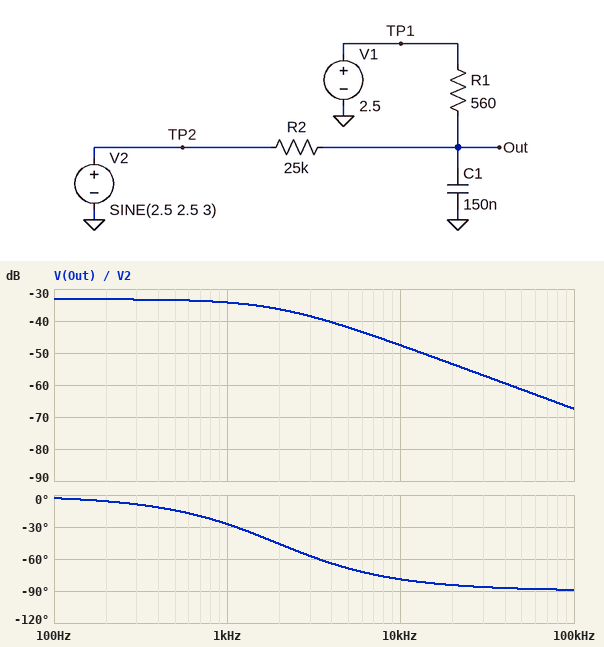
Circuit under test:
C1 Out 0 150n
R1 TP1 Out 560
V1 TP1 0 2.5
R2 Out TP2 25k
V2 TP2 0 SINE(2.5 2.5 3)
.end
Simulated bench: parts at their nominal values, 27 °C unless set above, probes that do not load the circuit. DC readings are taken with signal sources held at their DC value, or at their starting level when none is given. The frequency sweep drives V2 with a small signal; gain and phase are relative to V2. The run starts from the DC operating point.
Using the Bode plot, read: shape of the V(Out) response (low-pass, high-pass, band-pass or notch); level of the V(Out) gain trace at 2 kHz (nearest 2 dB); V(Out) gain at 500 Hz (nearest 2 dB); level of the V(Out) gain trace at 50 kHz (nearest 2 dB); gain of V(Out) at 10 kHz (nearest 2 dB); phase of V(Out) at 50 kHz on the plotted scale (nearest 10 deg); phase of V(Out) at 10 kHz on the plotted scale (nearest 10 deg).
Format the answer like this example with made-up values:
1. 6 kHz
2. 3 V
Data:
1. low-pass
2. -36 dB
3. -34 dB
4. -62 dB
5. -48 dB
6. -90 deg
7. -80 deg
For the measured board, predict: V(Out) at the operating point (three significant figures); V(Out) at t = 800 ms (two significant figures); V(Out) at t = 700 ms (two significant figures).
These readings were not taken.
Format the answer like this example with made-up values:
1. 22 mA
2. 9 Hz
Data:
1. 2.50 V
2. 2.5 V
3. 2.5 V
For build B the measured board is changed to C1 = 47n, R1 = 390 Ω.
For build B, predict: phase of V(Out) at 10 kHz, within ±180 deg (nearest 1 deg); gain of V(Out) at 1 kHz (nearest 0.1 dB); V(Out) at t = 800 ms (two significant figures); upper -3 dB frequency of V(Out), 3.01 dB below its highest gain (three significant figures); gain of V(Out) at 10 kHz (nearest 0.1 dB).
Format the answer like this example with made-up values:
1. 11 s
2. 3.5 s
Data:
1. -49 deg
2. -36.3 dB
3. 2.5 V
4. 8.82 kHz
5. -39.9 dB
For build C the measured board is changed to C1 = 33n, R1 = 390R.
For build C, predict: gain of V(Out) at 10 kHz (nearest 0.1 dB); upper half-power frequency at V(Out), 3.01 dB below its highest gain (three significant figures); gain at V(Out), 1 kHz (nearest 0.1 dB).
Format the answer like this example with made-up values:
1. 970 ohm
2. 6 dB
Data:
1. -38.4 dB
2. 12.6 kHz
3. -36.3 dB
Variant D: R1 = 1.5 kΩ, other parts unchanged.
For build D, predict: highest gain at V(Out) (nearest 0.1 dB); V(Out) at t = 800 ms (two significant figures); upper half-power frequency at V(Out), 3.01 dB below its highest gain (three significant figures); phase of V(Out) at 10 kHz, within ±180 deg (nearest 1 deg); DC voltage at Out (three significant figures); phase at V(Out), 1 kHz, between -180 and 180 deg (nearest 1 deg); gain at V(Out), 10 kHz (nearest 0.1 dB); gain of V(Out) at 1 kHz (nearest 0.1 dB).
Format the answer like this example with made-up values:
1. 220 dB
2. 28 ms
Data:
1. -24.9 dB
2. 2.6 V
3. 750 Hz
4. -86 deg
5. 2.50 V
6. -53 deg
7. -47.5 dB
8. -29.4 dB
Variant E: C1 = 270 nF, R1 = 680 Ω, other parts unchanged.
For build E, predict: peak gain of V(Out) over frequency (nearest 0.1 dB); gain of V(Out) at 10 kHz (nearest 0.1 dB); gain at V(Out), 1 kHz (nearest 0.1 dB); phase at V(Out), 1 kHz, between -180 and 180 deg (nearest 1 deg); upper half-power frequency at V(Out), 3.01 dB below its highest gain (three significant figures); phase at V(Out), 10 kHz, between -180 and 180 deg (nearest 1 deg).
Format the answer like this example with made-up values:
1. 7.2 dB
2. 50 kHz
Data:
1. -31.5 dB
2. -52.6 dB
3. -35.1 dB
4. -48 deg
5. 890 Hz
6. -85 deg
